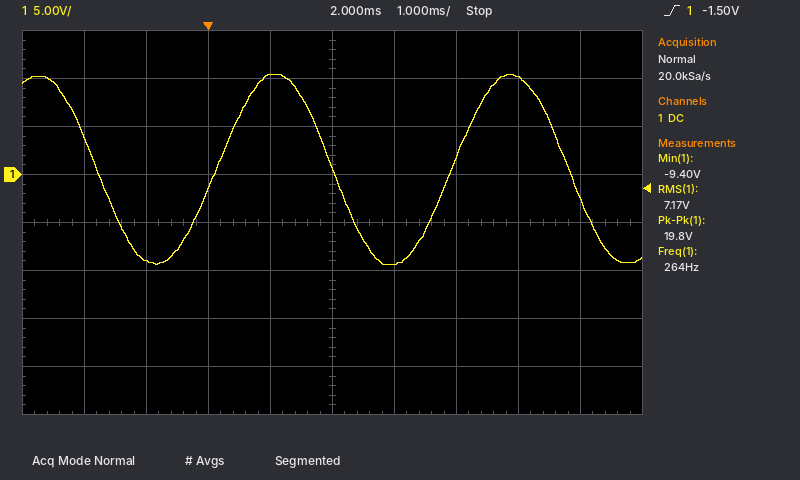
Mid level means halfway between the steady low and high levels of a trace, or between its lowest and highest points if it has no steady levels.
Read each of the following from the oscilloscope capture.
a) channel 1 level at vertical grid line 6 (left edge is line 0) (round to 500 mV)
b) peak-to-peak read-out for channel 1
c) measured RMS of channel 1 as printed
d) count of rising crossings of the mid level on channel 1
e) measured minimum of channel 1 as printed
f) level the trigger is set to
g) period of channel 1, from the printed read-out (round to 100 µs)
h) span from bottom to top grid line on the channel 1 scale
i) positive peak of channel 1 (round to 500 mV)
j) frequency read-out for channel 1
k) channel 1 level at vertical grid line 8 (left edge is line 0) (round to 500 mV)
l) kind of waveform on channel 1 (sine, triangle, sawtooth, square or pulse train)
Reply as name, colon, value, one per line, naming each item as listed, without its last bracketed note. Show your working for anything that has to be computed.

channel 1 level at vertical grid line 6 (left edge is line 0): -9.5 V
peak-to-peak read-out for channel 1: 19.8 V
measured RMS of channel 1 as printed: 7.17 V
count of rising crossings of the mid level on channel 1: 2
measured minimum of channel 1 as printed: -9.40 V
level the trigger is set to: -1.50 V
period of channel 1, from the printed read-out: 1 / 264 Hz ≈ 3.8 ms
span from bottom to top grid line on the channel 1 scale: 40 V
positive peak of channel 1: 10.5 V
frequency read-out for channel 1: 264 Hz
channel 1 level at vertical grid line 8 (left edge is line 0): 10.0 V
kind of waveform on channel 1: sine
